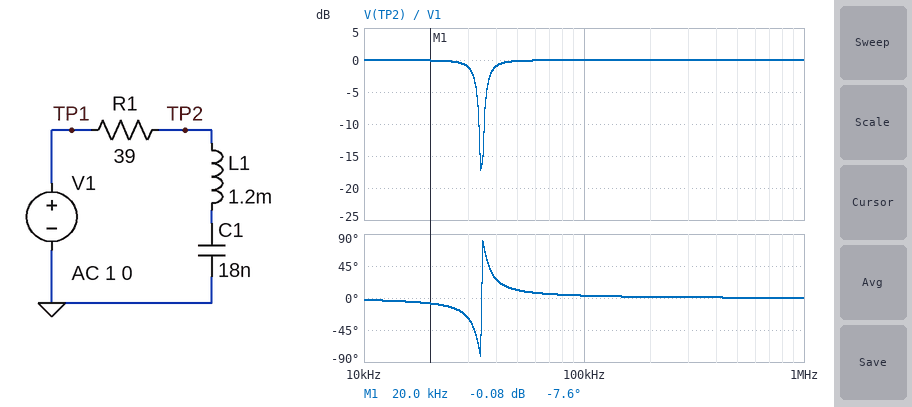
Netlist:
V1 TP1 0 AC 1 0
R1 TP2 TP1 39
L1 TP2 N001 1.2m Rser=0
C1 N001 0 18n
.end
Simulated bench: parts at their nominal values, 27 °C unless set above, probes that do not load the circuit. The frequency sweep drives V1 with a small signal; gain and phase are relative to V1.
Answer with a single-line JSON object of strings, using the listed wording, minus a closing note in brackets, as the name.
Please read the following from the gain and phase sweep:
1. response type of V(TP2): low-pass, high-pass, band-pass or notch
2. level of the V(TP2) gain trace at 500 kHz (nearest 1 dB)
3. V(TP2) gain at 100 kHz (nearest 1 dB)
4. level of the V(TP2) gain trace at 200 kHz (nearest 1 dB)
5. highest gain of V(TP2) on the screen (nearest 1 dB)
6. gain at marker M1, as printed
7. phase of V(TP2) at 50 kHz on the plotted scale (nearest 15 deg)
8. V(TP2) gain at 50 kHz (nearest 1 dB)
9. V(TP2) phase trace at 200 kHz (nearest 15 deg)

{"response type of V(TP2): low-pass, high-pass, band-pass or notch": "notch", "level of the V(TP2) gain trace at 500 kHz": "0 dB", "V(TP2) gain at 100 kHz": "0 dB", "level of the V(TP2) gain trace at 200 kHz": "0 dB", "highest gain of V(TP2) on the screen": "0 dB", "gain at marker M1, as printed": "-0.08 dB", "phase of V(TP2) at 50 kHz on the plotted scale": "15 deg", "V(TP2) gain at 50 kHz": "0 dB", "V(TP2) phase trace at 200 kHz": "0 deg"}
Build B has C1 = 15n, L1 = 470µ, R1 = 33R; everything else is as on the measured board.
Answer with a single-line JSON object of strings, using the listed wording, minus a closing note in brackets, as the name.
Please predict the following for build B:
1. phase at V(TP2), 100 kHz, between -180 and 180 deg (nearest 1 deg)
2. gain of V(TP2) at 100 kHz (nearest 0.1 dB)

{"phase at V(TP2), 100 kHz, between -180 and 180 deg": "10 deg", "gain of V(TP2) at 100 kHz": "-0.1 dB"}
